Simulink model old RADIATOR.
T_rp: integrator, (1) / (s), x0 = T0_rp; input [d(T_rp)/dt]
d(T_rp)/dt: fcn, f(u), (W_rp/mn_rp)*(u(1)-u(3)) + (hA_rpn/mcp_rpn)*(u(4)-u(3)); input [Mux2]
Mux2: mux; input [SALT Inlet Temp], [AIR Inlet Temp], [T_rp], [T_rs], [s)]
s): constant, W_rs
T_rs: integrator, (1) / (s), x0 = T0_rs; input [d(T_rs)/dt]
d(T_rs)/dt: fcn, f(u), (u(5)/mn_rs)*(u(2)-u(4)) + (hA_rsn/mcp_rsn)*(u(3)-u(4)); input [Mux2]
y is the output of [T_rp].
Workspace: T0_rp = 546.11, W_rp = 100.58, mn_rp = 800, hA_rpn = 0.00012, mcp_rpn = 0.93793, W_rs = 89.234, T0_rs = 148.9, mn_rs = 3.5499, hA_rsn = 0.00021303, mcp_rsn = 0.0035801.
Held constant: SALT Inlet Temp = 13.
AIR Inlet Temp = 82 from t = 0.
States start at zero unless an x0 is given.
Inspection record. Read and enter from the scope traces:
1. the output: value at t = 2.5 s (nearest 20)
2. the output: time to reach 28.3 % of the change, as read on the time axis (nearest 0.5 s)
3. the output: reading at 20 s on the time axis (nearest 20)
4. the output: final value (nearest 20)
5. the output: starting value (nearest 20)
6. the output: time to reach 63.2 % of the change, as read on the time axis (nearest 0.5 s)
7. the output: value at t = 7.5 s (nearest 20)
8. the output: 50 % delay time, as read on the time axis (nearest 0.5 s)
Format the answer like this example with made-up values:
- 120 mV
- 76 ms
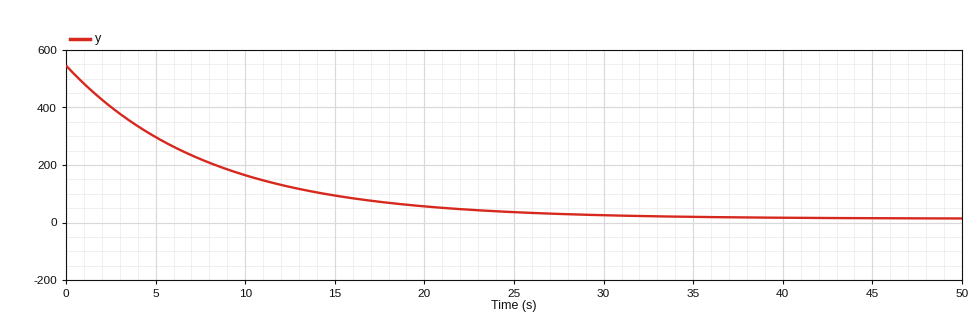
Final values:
- 400
- 2.5 s
- 60
- 20
- 540
- 8.0 s
- 220
- 5.5 s
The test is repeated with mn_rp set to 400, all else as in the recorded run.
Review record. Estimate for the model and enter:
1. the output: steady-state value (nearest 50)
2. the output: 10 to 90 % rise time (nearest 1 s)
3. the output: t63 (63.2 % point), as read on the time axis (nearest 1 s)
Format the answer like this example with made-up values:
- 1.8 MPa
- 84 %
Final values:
- 0
- 9 s
- 4 s
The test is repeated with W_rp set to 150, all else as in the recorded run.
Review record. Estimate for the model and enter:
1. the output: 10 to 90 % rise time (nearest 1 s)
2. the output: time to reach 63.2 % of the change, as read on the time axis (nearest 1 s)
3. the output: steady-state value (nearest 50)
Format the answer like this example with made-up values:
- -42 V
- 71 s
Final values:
- 12 s
- 5 s
- 0
